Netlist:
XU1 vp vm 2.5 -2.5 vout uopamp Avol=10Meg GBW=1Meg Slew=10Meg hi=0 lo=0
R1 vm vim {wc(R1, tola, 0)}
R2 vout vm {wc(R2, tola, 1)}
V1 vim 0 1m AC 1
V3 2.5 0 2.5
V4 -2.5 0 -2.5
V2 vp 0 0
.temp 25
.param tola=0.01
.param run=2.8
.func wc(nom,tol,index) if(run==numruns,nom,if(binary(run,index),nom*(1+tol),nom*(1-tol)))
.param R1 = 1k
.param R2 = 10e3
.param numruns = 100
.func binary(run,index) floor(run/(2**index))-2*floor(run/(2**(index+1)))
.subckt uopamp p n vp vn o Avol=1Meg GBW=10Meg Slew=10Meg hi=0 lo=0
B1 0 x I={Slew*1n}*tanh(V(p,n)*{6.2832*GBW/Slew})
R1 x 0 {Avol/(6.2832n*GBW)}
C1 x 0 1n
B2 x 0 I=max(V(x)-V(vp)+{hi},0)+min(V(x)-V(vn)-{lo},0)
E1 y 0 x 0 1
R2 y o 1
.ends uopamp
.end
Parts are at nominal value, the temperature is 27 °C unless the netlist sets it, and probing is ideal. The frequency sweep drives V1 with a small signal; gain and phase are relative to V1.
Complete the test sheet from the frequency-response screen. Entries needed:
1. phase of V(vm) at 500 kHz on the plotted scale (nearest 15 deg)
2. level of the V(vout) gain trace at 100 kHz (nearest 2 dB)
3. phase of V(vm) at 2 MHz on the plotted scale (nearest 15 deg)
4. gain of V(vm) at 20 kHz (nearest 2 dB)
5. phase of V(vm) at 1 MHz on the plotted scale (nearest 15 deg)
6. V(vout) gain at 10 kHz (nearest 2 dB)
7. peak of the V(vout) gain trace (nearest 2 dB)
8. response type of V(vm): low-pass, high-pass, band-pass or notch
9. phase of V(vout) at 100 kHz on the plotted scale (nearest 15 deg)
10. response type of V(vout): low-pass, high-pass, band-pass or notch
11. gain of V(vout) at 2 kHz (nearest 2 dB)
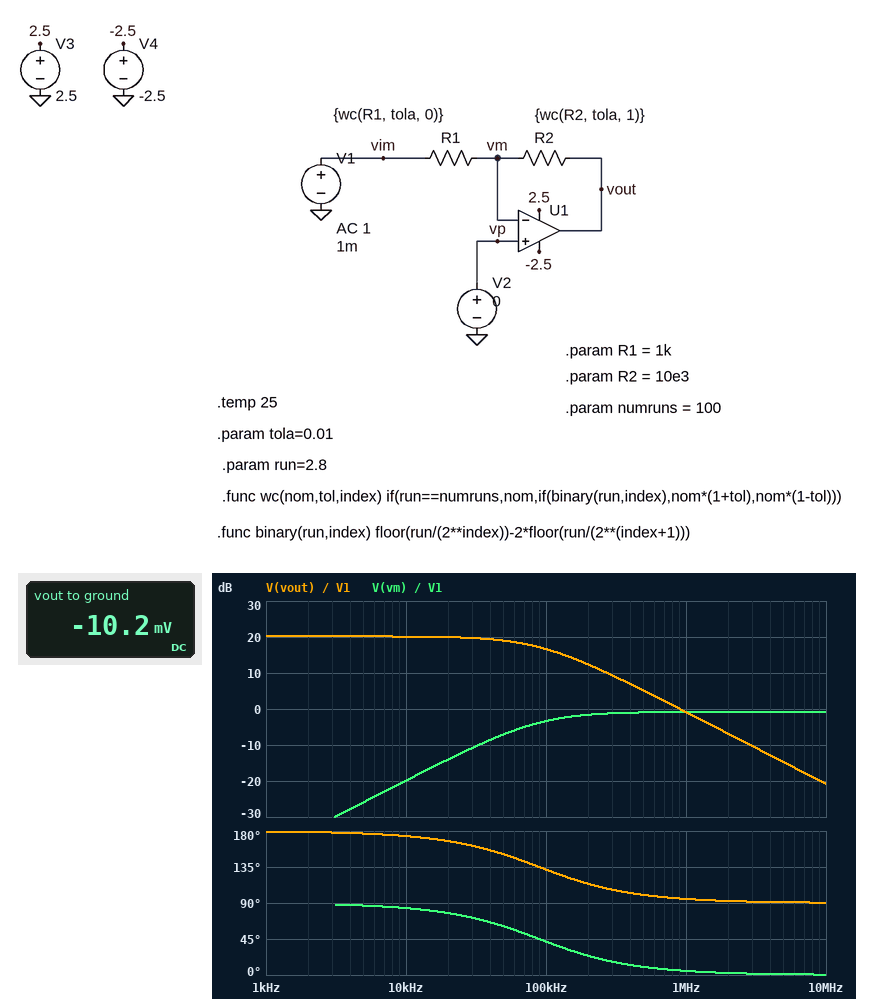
15 deg
16 dB
0 deg
-14 dB
0 deg
20 dB
20 dB
high-pass
135 deg
low-pass
20 dB
